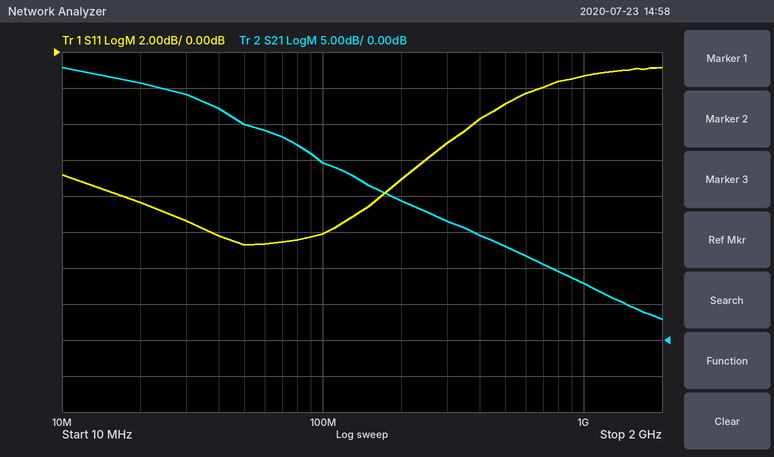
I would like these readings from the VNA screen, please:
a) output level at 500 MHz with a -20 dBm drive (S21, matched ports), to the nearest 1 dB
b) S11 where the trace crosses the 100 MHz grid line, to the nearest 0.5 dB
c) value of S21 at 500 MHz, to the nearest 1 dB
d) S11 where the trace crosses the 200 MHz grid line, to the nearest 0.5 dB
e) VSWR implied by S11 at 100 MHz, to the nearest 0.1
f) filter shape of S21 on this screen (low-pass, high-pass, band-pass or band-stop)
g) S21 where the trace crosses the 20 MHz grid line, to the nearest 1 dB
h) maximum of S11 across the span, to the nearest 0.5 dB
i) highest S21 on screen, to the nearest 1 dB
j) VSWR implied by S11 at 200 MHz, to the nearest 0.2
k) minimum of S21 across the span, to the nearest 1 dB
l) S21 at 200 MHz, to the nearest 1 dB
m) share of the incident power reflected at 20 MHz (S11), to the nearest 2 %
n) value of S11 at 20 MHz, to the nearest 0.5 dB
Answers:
-7 dBm
-10.0 dB
13 dB
-7.0 dB
1.9
low-pass
36 dB
-1.0 dB
38 dB
2.6
3 dB
19 dB
14 %
-8.5 dB
